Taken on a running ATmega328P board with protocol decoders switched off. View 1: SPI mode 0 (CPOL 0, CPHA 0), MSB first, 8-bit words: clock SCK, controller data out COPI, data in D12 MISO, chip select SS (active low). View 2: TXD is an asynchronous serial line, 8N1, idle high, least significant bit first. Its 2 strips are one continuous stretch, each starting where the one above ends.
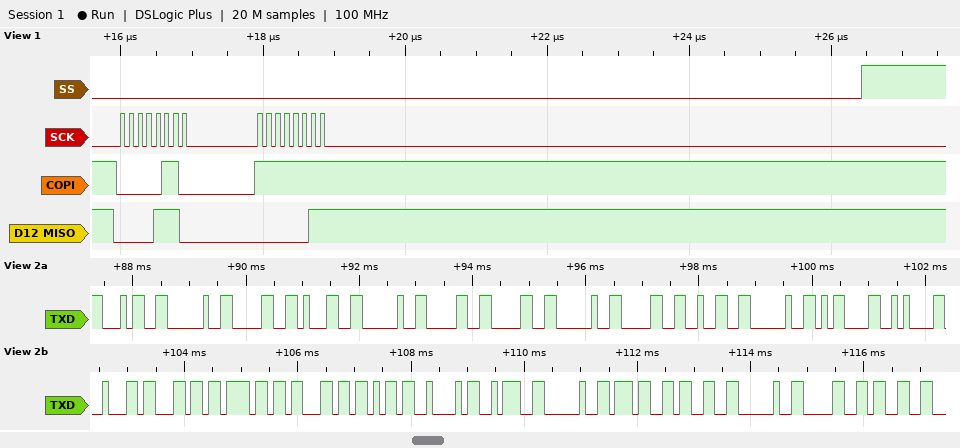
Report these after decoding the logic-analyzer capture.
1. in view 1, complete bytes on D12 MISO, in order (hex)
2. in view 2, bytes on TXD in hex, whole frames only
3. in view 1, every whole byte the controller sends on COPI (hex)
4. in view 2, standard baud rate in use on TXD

0x0E 0x03
34 20 30 31 20 30 30 20 30 32 20 0D 0A 62 6C 6F 63 6B 42 3A 20 37 33 20 30 33
0x06 0xFF
9600 baud
